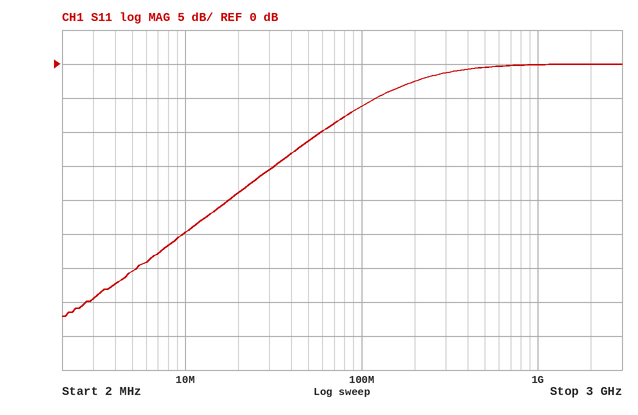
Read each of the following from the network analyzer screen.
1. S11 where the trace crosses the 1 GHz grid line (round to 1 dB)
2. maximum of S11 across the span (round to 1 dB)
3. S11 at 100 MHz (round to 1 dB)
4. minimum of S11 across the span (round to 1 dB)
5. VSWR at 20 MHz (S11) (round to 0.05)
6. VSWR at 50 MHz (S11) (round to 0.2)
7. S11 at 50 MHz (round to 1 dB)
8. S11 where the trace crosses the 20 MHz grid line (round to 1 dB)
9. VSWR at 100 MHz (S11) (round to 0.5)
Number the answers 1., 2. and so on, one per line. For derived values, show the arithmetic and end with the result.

1. 0 dB
2. 0 dB
3. -6 dB
4. -37 dB
5. |Γ| = 10^(-19/20) = 0.1122; VSWR = (1 + 0.1122)/(1 − 0.1122) ≈ 1.25
6. |Γ| = 10^(-11/20) = 0.2818; VSWR = (1 + 0.2818)/(1 − 0.2818) ≈ 1.8
7. -11 dB
8. -19 dB
9. |Γ| = 10^(-6/20) = 0.5012; VSWR = (1 + 0.5012)/(1 − 0.5012) ≈ 3.0
